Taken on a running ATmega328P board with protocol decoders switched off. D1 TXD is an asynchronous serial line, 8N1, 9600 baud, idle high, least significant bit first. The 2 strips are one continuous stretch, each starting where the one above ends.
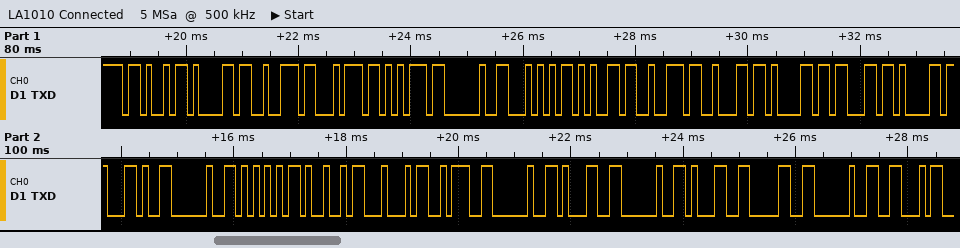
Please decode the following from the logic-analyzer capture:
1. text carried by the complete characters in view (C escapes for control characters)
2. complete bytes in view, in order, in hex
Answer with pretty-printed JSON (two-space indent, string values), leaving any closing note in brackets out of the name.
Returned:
{
  "text carried by the complete characters in view": "\"Kartu Terbaca, UID: 1 10 F\"",
  "complete bytes in view, in order, in hex": "4B 61 72 74 75 20 54 65 72 62 61 63 61 2C 20 55 49 44 3A 20 31 20 31 30 20 46"
}
